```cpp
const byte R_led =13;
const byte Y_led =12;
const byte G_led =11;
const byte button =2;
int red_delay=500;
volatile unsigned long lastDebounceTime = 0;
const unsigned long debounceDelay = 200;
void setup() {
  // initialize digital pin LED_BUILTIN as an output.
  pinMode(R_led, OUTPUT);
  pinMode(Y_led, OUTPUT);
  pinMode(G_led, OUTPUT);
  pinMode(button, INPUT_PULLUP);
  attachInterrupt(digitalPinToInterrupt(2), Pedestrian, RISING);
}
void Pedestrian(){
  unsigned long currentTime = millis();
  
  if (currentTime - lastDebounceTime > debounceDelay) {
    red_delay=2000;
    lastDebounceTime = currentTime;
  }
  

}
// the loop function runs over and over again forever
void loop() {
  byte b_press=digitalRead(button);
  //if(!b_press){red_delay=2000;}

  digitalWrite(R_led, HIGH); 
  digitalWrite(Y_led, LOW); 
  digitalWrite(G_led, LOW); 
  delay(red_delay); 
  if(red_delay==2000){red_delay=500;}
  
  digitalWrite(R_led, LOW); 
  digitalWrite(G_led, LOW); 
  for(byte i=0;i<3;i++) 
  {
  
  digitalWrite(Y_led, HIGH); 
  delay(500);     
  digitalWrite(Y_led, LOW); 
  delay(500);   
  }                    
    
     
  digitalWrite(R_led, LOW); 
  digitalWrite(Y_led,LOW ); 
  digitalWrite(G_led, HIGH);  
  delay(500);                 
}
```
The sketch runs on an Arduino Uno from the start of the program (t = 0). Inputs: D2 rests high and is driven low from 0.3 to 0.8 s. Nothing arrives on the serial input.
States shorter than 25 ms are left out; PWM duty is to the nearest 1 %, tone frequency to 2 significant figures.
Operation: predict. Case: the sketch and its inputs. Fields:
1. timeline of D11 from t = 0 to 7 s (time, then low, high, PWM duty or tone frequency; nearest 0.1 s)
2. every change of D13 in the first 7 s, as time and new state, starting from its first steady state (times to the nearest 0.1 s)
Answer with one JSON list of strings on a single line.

["0 s low; 3.5 s high; 4 s low", "0 s high; 0.5 s low; 4 s high; 6 s low"]
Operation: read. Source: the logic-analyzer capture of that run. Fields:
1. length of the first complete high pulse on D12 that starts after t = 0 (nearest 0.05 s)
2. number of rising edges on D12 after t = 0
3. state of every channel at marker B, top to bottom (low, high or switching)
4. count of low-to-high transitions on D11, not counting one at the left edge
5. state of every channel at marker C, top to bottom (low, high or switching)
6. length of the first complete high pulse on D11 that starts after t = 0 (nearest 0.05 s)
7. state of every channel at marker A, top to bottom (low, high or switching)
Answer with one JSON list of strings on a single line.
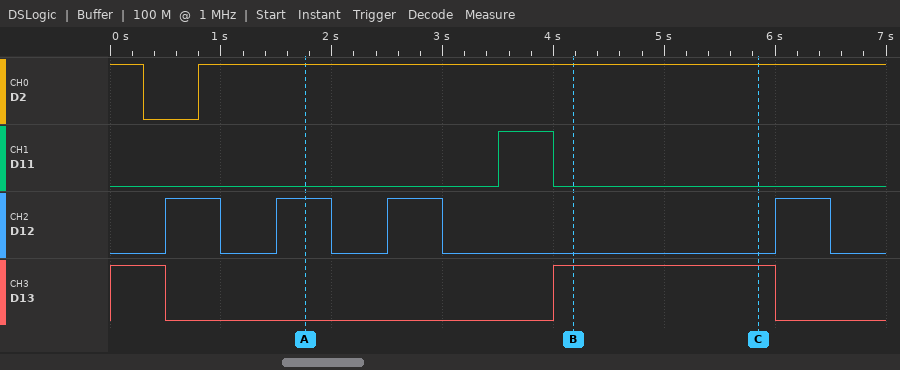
["0.50 s", "4", "D2 high, D11 low, D12 low, D13 high", "1", "D2 high, D11 low, D12 low, D13 high", "0.50 s", "D2 high, D11 low, D12 high, D13 low"]
